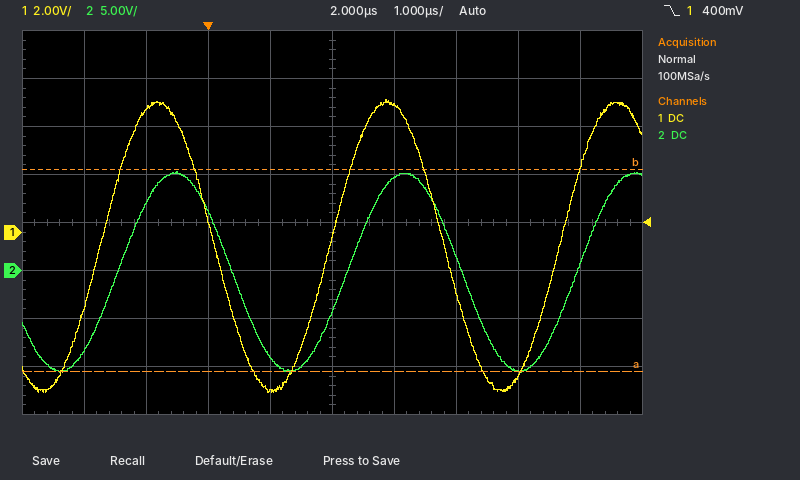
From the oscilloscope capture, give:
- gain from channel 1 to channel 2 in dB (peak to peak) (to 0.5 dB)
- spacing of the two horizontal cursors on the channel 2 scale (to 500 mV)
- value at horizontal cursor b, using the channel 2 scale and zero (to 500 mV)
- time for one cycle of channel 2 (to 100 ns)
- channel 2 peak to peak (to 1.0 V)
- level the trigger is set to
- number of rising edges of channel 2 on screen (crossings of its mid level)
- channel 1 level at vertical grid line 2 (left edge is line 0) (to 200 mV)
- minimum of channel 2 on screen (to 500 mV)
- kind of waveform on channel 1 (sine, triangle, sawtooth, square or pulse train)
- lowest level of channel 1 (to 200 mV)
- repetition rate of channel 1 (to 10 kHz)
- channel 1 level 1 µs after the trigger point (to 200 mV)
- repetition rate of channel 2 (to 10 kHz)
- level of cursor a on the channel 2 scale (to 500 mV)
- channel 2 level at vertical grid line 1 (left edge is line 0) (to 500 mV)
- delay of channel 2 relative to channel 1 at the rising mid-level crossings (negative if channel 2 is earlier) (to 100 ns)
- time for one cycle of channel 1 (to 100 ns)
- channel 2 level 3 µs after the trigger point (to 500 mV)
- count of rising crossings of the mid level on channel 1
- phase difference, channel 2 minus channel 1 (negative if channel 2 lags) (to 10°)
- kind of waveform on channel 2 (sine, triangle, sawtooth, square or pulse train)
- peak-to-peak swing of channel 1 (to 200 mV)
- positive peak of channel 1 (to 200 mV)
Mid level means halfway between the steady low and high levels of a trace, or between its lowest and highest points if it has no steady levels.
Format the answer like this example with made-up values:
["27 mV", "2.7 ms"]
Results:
["4.5 dB", "21.0 V", "10.5 V", "3.7 µs", "21.0 V", "400 mV", "3", "5.0 V", "-10.5 V", "sine", "-6.6 V", "270 kHz", "-6.6 V", "270 kHz", "-10.5 V", "-8.5 V", "+300 ns", "3.7 µs", "9.5 V", "3", "-30°", "sine", "12.2 V", "5.6 V"]
